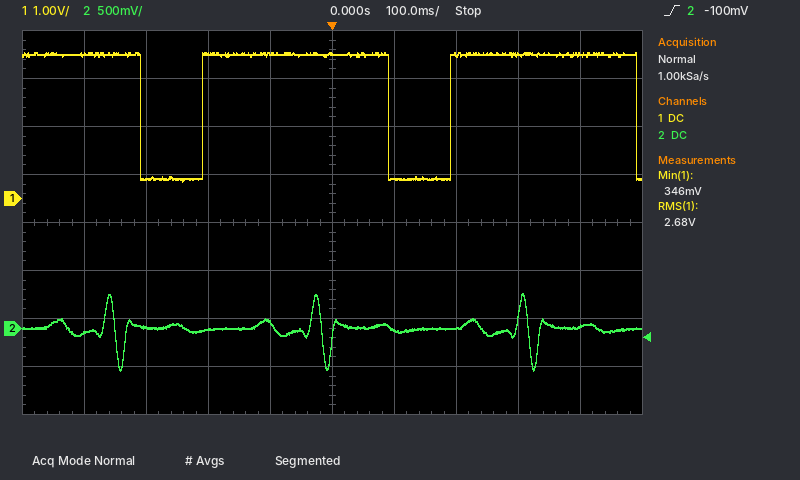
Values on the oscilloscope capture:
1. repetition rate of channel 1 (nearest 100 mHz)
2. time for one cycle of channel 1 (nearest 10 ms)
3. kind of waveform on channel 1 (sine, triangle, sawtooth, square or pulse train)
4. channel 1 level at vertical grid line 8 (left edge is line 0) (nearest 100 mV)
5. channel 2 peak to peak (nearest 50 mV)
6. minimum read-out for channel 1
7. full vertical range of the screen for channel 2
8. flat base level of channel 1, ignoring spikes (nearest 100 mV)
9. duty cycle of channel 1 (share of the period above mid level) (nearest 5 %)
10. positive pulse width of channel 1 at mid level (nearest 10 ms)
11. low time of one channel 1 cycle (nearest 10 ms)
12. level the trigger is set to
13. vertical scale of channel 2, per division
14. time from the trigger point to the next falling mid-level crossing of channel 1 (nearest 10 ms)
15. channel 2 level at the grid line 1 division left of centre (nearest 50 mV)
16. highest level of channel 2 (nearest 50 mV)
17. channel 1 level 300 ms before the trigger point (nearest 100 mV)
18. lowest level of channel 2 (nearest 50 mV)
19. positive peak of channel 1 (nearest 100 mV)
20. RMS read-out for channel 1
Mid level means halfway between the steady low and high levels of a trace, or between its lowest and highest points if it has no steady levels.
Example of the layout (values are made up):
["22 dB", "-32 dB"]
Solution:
["2.5 Hz", "400 ms", "pulse train", "3.0 V", "800 mV", "346 mV", "4 V", "400 mV", "75 %", "300 ms", "100 ms", "-100 mV", "500 mV", "90 ms", "50 mV", "350 mV", "400 mV", "-450 mV", "3.0 V", "2.68 V"]
